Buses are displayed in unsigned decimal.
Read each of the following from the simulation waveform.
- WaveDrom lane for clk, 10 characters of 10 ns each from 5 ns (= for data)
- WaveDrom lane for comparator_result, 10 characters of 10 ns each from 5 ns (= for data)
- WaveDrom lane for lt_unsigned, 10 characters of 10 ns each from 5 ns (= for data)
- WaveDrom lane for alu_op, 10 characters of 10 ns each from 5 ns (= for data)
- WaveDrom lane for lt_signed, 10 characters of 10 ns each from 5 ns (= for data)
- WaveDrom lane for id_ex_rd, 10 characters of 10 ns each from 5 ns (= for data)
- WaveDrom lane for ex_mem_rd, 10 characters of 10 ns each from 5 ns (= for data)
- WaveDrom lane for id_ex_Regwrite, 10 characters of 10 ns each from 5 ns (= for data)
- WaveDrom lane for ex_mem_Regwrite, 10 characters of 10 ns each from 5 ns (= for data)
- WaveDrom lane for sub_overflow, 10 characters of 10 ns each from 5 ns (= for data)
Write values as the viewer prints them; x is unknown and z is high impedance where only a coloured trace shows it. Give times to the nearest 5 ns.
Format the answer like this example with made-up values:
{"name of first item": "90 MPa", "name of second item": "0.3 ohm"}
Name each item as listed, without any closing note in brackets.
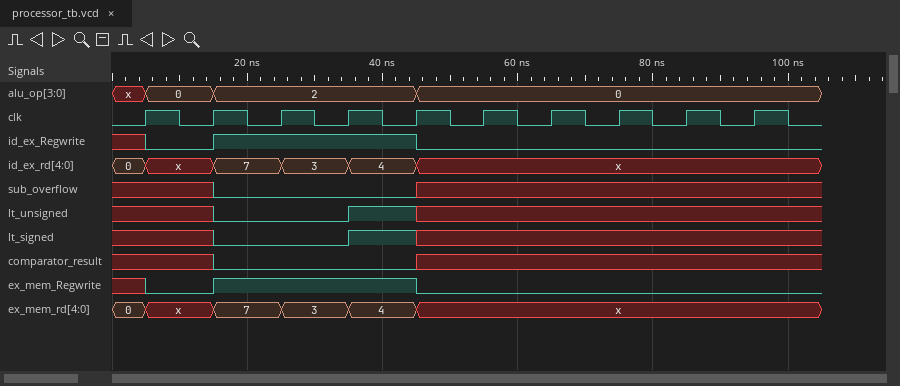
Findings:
{"WaveDrom lane for clk, 10 characters of 10 ns each from 5 ns": "{name: 'clk', wave: 'p.........'}", "WaveDrom lane for comparator_result, 10 characters of 10 ns each from 5 ns": "{name: 'comparator_result', wave: 'x0..x.....'}", "WaveDrom lane for lt_unsigned, 10 characters of 10 ns each from 5 ns": "{name: 'lt_unsigned', wave: 'x0.1x.....'}", "WaveDrom lane for alu_op, 10 characters of 10 ns each from 5 ns": "{name: 'alu_op', wave: '==..=.....', data: '0 2 0'}", "WaveDrom lane for lt_signed, 10 characters of 10 ns each from 5 ns": "{name: 'lt_signed', wave: 'x0.1x.....'}", "WaveDrom lane for id_ex_rd, 10 characters of 10 ns each from 5 ns": "{name: 'id_ex_rd', wave: 'x===x.....', data: '7 3 4'}", "WaveDrom lane for ex_mem_rd, 10 characters of 10 ns each from 5 ns": "{name: 'ex_mem_rd', wave: 'x===x.....', data: '7 3 4'}", "WaveDrom lane for id_ex_Regwrite, 10 characters of 10 ns each from 5 ns": "{name: 'id_ex_Regwrite', wave: '01..0.....'}", "WaveDrom lane for ex_mem_Regwrite, 10 characters of 10 ns each from 5 ns": "{name: 'ex_mem_Regwrite', wave: '01..0.....'}", "WaveDrom lane for sub_overflow, 10 characters of 10 ns each from 5 ns": "{name: 'sub_overflow', wave: 'x0..x.....'}"}
